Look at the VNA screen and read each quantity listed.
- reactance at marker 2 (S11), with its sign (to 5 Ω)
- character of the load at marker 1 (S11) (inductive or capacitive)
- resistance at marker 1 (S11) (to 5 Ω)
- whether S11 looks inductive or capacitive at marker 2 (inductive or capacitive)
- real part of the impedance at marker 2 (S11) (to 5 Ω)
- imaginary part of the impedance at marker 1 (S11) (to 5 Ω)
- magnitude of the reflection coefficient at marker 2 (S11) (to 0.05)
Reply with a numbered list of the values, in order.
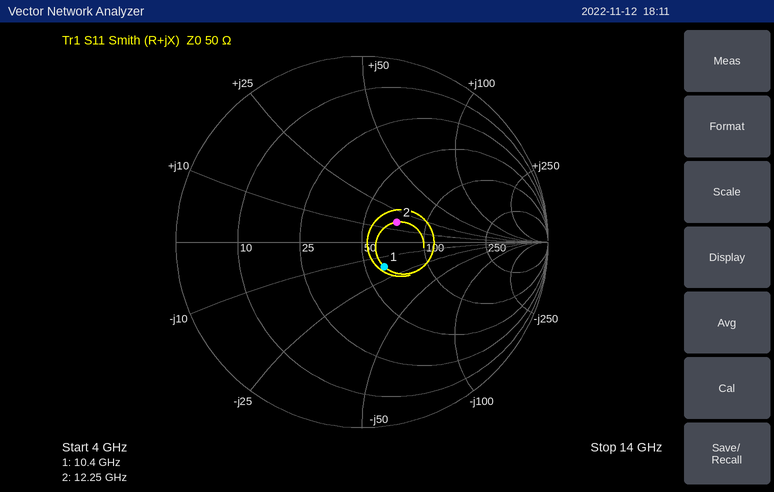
1. +15 Ω
2. capacitive
3. 60 Ω
4. inductive
5. 70 Ω
6. -15 Ω
7. 0.20
